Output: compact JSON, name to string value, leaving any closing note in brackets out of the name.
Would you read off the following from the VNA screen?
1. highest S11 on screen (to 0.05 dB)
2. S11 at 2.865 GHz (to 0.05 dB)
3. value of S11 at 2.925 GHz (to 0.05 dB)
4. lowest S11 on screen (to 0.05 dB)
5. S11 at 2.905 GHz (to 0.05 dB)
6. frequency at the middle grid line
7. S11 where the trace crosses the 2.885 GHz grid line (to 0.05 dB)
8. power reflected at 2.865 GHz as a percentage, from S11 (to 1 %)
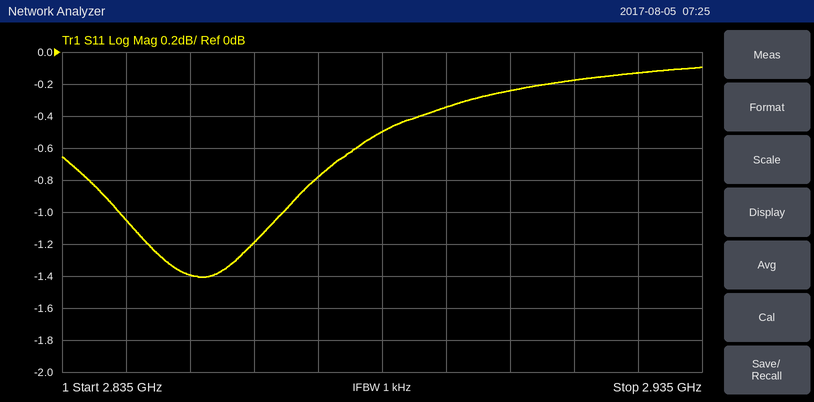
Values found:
{"highest S11 on screen": "-0.10 dB", "S11 at 2.865 GHz": "-1.20 dB", "value of S11 at 2.925 GHz": "-0.15 dB", "lowest S11 on screen": "-1.40 dB", "S11 at 2.905 GHz": "-0.25 dB", "frequency at the middle grid line": "2.885 GHz", "S11 where the trace crosses the 2.885 GHz grid line": "-0.50 dB", "power reflected at 2.865 GHz as a percentage, from S11": "76 %"}
